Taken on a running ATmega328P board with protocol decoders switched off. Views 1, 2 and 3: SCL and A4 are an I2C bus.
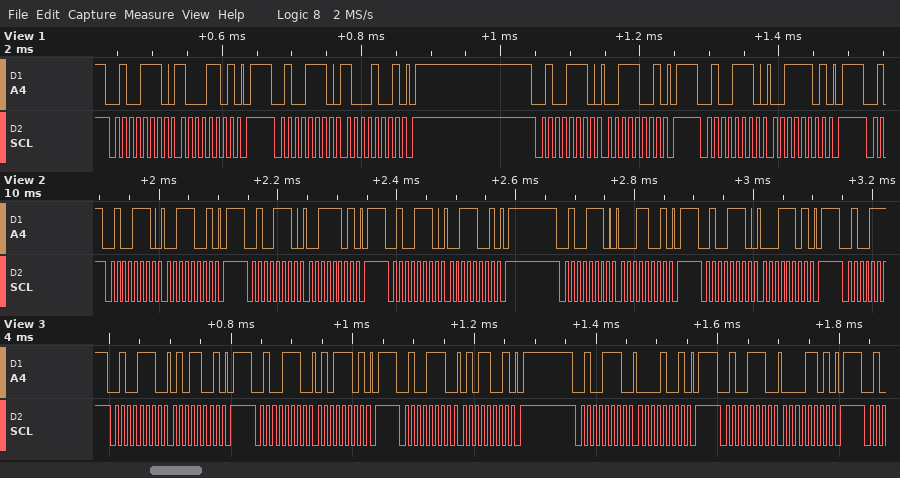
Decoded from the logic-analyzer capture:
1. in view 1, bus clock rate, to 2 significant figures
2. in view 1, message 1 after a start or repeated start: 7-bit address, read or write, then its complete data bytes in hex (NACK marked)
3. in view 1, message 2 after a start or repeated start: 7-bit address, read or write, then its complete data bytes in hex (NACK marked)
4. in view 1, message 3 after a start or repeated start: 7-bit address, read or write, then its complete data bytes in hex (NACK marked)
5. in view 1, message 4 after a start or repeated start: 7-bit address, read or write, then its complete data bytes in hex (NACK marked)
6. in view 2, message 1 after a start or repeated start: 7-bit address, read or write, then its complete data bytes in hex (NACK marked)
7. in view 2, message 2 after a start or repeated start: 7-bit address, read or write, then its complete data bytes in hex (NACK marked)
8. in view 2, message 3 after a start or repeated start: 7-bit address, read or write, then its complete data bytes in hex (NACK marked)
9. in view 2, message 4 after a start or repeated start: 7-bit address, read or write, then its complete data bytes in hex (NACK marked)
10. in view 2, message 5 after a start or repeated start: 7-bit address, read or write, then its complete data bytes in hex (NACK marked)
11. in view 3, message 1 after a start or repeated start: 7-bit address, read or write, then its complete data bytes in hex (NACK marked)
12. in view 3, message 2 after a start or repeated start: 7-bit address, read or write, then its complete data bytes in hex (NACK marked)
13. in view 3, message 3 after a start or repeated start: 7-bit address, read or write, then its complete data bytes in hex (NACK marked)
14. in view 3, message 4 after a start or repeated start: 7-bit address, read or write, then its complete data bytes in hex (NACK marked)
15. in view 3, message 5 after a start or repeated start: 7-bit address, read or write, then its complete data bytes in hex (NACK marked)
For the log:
100 kHz
0x27 write: 8D
0x27 write: 89
0x27 write: 39
0x27 write: 3D
0x27 write: 39
0x27 write: 3D
0x27 write: 39
0x27 write: 19
0x27 write: 1D
0x27 write: 59
0x27 write: 5D
0x27 write: 59
0x27 write: 09
0x27 write: 0D
